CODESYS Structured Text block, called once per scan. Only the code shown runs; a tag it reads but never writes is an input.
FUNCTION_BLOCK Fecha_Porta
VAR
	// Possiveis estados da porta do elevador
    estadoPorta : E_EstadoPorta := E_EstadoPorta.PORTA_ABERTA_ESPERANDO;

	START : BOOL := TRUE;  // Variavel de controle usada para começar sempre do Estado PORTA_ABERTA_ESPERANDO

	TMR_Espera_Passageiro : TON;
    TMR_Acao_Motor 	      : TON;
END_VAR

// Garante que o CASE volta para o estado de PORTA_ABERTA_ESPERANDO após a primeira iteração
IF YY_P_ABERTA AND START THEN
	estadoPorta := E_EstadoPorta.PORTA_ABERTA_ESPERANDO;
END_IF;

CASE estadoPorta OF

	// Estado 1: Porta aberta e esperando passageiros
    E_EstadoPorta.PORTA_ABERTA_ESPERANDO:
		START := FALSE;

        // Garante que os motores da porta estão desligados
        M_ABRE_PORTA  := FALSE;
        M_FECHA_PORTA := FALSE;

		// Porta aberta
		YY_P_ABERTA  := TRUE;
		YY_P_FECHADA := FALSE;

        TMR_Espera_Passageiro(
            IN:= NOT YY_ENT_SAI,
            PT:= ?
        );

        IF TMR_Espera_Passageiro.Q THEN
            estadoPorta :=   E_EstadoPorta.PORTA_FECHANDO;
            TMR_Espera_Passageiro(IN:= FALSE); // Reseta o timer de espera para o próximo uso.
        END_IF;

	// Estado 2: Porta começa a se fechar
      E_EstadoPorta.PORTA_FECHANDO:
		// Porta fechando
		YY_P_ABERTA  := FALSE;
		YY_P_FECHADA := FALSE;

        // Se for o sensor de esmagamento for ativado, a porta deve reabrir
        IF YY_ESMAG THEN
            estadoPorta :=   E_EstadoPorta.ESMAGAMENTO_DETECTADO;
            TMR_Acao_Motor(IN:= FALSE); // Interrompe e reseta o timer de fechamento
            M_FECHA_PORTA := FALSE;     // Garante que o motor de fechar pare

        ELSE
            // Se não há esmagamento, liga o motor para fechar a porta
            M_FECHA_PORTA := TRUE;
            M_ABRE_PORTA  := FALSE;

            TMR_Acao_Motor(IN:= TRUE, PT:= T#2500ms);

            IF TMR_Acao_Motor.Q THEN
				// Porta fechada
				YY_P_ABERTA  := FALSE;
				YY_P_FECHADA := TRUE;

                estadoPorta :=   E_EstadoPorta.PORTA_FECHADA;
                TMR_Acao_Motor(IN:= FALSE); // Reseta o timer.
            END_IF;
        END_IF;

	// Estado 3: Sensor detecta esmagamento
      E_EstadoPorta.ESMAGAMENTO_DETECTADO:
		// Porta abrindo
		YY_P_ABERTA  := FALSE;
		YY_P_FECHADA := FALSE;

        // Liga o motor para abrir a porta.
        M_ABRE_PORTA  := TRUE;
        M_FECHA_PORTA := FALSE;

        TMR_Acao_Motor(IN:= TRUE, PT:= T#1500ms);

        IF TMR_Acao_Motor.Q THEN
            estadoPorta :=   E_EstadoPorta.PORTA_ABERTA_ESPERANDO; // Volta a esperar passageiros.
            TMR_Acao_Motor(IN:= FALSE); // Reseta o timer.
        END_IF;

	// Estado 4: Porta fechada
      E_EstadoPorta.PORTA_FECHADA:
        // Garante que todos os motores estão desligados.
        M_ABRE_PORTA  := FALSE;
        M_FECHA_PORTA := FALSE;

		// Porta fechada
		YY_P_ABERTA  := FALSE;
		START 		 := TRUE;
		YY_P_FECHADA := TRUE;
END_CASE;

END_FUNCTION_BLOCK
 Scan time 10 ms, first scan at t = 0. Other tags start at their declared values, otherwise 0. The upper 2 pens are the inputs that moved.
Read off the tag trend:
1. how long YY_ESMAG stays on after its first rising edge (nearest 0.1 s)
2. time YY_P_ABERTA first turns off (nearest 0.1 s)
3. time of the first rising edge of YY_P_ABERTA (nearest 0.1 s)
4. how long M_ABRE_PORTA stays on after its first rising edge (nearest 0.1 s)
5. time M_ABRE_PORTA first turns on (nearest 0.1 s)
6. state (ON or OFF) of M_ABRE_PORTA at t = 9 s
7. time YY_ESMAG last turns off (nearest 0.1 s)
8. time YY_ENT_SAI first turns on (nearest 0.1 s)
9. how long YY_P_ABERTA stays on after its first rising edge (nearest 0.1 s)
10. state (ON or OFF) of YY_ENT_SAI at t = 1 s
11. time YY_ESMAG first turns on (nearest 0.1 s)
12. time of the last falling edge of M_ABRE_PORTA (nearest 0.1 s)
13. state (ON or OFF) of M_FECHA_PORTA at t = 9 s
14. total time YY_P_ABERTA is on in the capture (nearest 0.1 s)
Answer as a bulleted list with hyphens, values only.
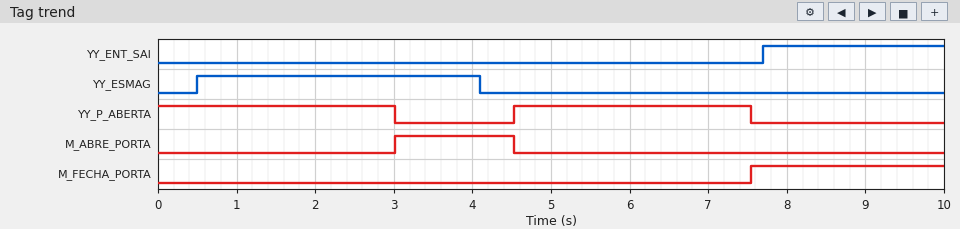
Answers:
- 3.6 s
- 3.0 s
- 4.5 s
- 1.5 s
- 3.0 s
- OFF
- 4.1 s
- 7.7 s
- 3.0 s
- OFF
- 0.5 s
- 4.5 s
- ON
- 6.0 s
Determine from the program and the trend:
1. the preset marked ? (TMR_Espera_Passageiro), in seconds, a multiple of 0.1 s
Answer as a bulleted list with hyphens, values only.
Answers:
- 3.0 s
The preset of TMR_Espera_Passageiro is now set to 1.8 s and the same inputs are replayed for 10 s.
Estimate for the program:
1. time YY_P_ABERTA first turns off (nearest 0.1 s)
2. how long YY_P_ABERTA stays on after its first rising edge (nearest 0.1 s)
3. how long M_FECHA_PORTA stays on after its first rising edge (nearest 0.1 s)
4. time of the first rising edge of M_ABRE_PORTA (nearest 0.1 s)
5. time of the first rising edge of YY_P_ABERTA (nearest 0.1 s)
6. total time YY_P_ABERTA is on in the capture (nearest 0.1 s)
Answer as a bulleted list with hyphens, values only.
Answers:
- 1.8 s
- 1.8 s
- 2.5 s
- 1.8 s
- 3.3 s
- 3.6 s
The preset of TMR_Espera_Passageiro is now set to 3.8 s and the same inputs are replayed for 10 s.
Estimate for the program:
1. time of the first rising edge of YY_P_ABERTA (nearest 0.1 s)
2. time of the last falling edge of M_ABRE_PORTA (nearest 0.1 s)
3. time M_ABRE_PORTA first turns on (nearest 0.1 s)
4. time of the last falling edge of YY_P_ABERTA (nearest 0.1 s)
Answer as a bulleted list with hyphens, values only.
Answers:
- 5.3 s
- 5.3 s
- 3.8 s
- 3.8 s
